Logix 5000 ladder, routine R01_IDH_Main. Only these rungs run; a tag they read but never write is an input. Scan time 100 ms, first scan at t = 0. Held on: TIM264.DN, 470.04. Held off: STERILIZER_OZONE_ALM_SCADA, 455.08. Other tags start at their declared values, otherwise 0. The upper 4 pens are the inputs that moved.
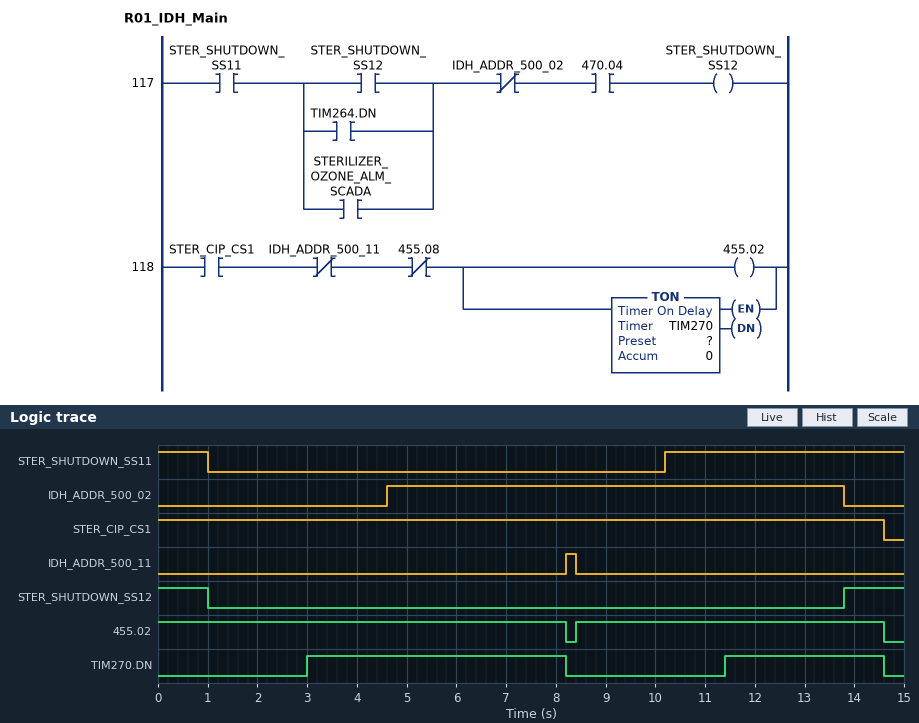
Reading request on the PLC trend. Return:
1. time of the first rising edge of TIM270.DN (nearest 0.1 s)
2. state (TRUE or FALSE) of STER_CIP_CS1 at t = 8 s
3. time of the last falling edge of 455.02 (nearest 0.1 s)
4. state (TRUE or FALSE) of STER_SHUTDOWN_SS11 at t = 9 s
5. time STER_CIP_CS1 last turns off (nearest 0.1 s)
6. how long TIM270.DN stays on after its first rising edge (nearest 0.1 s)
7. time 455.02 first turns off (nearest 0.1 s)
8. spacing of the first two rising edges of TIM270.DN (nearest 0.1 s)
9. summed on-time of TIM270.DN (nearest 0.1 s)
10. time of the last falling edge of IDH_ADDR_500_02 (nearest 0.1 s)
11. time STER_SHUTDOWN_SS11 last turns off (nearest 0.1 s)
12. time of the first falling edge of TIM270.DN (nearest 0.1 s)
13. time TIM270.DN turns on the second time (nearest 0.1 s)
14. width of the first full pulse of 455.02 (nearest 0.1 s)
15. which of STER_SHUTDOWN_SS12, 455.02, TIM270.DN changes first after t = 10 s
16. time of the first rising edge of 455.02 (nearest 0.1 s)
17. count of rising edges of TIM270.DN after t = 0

3.0 s
TRUE
14.6 s
FALSE
14.6 s
5.2 s
8.2 s
8.4 s
8.4 s
13.8 s
1.0 s
8.2 s
11.4 s
6.2 s
TIM270.DN
8.4 s
2
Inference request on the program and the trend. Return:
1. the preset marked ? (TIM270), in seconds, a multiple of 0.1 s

3.0 s
